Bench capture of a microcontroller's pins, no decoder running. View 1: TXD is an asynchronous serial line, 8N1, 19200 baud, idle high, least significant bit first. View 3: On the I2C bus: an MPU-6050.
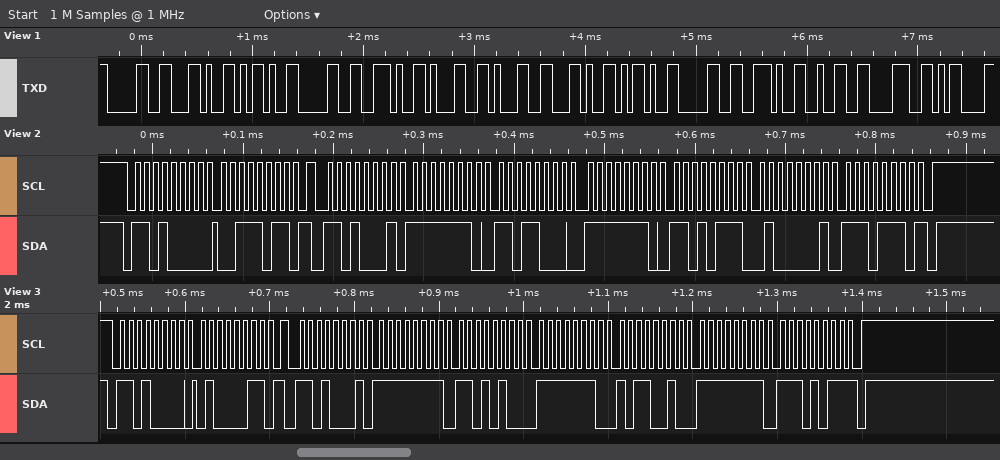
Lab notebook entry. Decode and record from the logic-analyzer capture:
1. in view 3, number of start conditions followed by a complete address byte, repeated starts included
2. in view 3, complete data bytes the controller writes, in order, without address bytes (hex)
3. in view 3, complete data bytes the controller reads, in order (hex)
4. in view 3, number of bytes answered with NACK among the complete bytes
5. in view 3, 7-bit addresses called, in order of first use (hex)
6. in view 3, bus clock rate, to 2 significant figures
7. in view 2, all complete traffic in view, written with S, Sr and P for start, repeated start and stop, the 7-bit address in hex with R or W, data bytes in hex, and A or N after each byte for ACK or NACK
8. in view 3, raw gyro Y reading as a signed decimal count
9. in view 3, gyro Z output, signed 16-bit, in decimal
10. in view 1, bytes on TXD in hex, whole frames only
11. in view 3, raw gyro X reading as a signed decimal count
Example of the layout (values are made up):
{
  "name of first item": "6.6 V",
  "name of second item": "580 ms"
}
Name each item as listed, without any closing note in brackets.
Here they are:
{
  "in view 3, number of start conditions followed by a complete address byte, repeated starts included": "2",
  "in view 3, complete data bytes the controller writes, in order, without address bytes": "43",
  "in view 3, complete data bytes the controller reads, in order": "FF D4 FE B2 FF EB",
  "in view 3, number of bytes answered with NACK among the complete bytes": "1",
  "in view 3, 7-bit addresses called, in order of first use": "0x68",
  "in view 3, bus clock rate, to 2 significant figures": "100 kHz",
  "in view 2, all complete traffic in view, written with S, Sr and P for start, repeated start and stop, the 7-bit address in hex with R or W, data bytes in hex, and A or N after each byte for ACK or NACK": "S 68W A 3B A Sr 68R A FE A D8 A FE A D7 A 41 A EE N P",
  "in view 3, raw gyro Y reading as a signed decimal count": "-334",
  "in view 3, gyro Z output, signed 16-bit, in decimal": "-21",
  "in view 1, bytes on TXD in hex, whole frames only": "30 2C 2D 30 2E 31 31 2C 2D 30 2E 32 38 0D",
  "in view 3, raw gyro X reading as a signed decimal count": "-44"
}
